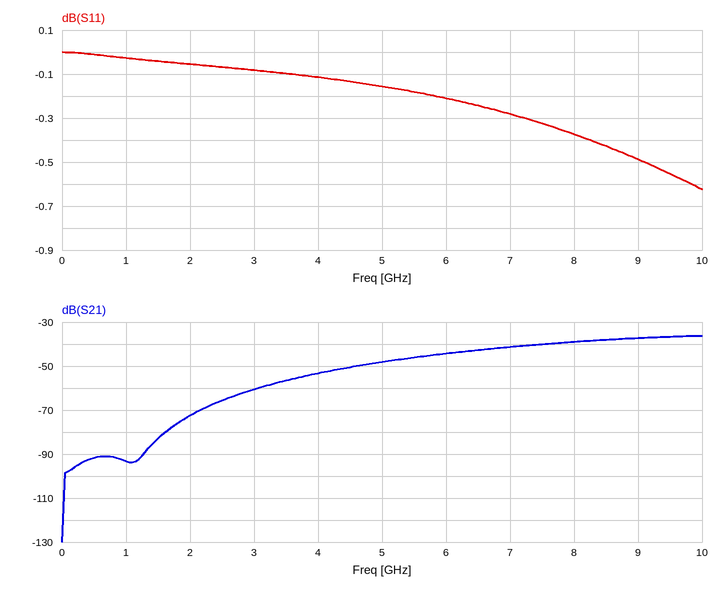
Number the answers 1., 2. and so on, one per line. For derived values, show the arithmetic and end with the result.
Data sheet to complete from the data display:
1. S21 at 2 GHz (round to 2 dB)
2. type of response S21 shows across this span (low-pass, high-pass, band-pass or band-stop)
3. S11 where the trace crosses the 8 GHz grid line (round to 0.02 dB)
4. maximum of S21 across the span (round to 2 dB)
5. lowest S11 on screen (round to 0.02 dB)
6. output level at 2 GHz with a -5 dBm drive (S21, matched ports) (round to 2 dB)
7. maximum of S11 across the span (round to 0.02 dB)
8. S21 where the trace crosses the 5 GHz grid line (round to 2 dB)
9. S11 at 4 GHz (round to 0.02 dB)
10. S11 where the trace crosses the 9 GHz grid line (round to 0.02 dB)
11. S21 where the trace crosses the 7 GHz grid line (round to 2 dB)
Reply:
1. -72 dB
2. high-pass
3. -0.38 dB
4. -36 dB
5. -0.62 dB
6. -5 dBm + (-72 dB) = -78 dBm
7. 0.00 dB
8. -48 dB
9. -0.12 dB
10. -0.48 dB
11. -42 dB
